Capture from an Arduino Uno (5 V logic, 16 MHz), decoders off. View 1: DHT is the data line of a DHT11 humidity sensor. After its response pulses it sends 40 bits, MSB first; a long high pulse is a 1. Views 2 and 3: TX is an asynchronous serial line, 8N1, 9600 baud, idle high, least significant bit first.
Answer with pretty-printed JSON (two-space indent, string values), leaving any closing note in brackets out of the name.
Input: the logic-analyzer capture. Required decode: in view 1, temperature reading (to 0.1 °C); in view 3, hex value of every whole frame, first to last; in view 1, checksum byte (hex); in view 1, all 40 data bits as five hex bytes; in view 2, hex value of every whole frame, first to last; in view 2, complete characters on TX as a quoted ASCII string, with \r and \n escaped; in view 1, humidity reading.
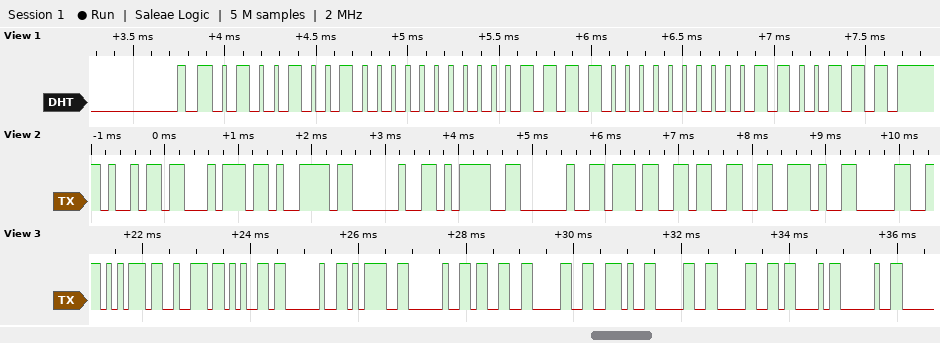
{
  "in view 1, temperature reading": "30.0 °C",
  "in view 3, hex value of every whole frame, first to last": "75 72 65 20 3D 20 33 30 2E 30 30 43 20",
  "in view 1, checksum byte": "0x67",
  "in view 1, all 40 data bits as five hex bytes": "49 00 1E 00 67",
  "in view 2, hex value of every whole frame, first to last": "69 74 79 20 3D 20 37 33 2E 30",
  "in view 2, complete characters on TX as a quoted ASCII string, with \\r and \\n escaped": "\"ity = 73.0\"",
  "in view 1, humidity reading": "73 %"
}
